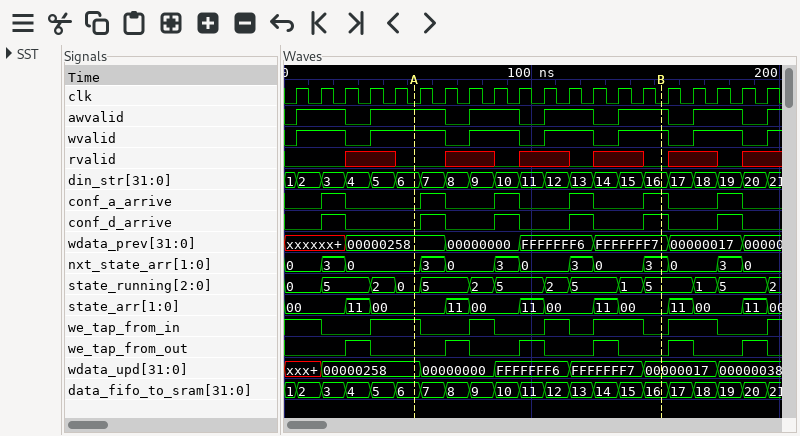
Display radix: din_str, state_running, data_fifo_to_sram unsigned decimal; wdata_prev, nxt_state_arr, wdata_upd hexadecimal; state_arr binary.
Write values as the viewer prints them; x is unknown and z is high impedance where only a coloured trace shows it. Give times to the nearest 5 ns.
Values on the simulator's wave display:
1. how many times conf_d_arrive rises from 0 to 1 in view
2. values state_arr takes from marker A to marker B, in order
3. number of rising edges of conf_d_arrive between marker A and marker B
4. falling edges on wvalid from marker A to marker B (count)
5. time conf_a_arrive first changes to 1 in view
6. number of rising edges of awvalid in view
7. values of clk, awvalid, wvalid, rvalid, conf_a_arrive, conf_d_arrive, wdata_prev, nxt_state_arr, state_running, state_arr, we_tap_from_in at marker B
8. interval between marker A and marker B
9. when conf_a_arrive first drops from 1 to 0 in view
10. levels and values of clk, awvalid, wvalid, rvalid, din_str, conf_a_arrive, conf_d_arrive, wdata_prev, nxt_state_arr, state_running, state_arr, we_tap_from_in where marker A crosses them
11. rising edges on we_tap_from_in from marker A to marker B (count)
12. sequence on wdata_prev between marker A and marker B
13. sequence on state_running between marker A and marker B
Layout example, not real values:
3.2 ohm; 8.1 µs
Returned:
6; 00, 11, 00, 11, 00, 11, 00; 4; 3; 15 ns; 7; clk=0, awvalid=1, wvalid=1, rvalid=0, conf_a_arrive=1, conf_d_arrive=1, wdata_prev=FFFFFFF7, nxt_state_arr=3, state_running=5, state_arr=00, we_tap_from_in=0; 100 ns; 25 ns; clk=0, awvalid=1, wvalid=1, rvalid=0, din_str=6, conf_a_arrive=0, conf_d_arrive=0, wdata_prev=00000258, nxt_state_arr=0, state_running=0, state_arr=00, we_tap_from_in=1; 3; 00000258, 00000000, FFFFFFF6, FFFFFFF7; 0, 5, 2, 5, 2, 5, 1, 5
